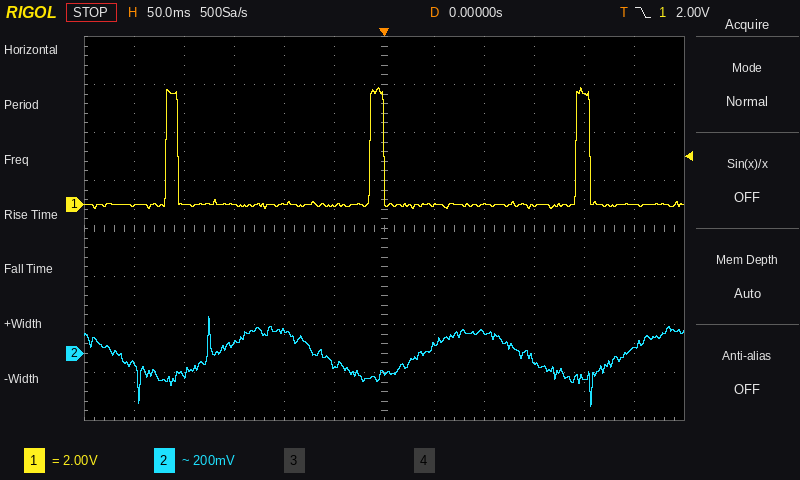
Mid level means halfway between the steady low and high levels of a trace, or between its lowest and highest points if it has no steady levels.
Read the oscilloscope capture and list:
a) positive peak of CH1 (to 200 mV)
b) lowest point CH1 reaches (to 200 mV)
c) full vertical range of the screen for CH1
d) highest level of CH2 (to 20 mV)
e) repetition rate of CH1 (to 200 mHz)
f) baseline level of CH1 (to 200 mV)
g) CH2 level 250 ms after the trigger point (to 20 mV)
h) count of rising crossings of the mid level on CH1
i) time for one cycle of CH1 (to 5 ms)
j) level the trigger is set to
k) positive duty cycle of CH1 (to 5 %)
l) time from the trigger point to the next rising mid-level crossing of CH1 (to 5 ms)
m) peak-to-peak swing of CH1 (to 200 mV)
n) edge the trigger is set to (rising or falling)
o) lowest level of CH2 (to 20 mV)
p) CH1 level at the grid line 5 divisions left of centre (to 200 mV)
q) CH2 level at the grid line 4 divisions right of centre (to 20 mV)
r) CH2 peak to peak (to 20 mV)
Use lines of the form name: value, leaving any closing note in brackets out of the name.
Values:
positive peak of CH1: 4.8 V
lowest point CH1 reaches: -200 mV
full vertical range of the screen for CH1: 16 V
highest level of CH2: 160 mV
repetition rate of CH1: 4.8 Hz
baseline level of CH1: 0.0 V
CH2 level 250 ms after the trigger point: 20 mV
count of rising crossings of the mid level on CH1: 3
time for one cycle of CH1: 205 ms
level the trigger is set to: 2.00 V
positive duty cycle of CH1: 5 %
time from the trigger point to the next rising mid-level crossing of CH1: 190 ms
peak-to-peak swing of CH1: 5.0 V
edge the trigger is set to: falling
lowest level of CH2: -220 mV
CH1 level at the grid line 5 divisions left of centre: 0.0 V
CH2 level at the grid line 4 divisions right of centre: -100 mV
CH2 peak to peak: 380 mV
